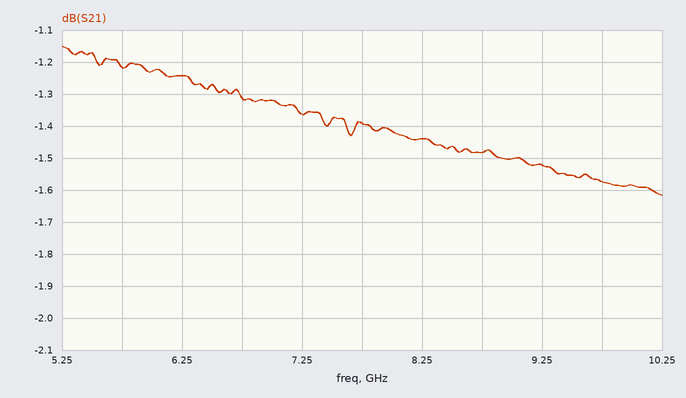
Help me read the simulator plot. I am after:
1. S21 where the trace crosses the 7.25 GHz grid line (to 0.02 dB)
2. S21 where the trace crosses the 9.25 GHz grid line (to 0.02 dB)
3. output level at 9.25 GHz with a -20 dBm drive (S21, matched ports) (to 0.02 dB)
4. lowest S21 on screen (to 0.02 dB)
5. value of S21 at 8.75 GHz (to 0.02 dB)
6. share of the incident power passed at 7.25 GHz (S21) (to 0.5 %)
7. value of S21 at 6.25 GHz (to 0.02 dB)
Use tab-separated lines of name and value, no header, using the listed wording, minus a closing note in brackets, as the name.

S21 where the trace crosses the 7.25 GHz grid line	-1.36 dB
S21 where the trace crosses the 9.25 GHz grid line	-1.52 dB
output level at 9.25 GHz with a -20 dBm drive (S21, matched ports)	-21.52 dBm
lowest S21 on screen	-1.62 dB
value of S21 at 8.75 GHz	-1.48 dB
share of the incident power passed at 7.25 GHz (S21)	73.0 %
value of S21 at 6.25 GHz	-1.24 dB
